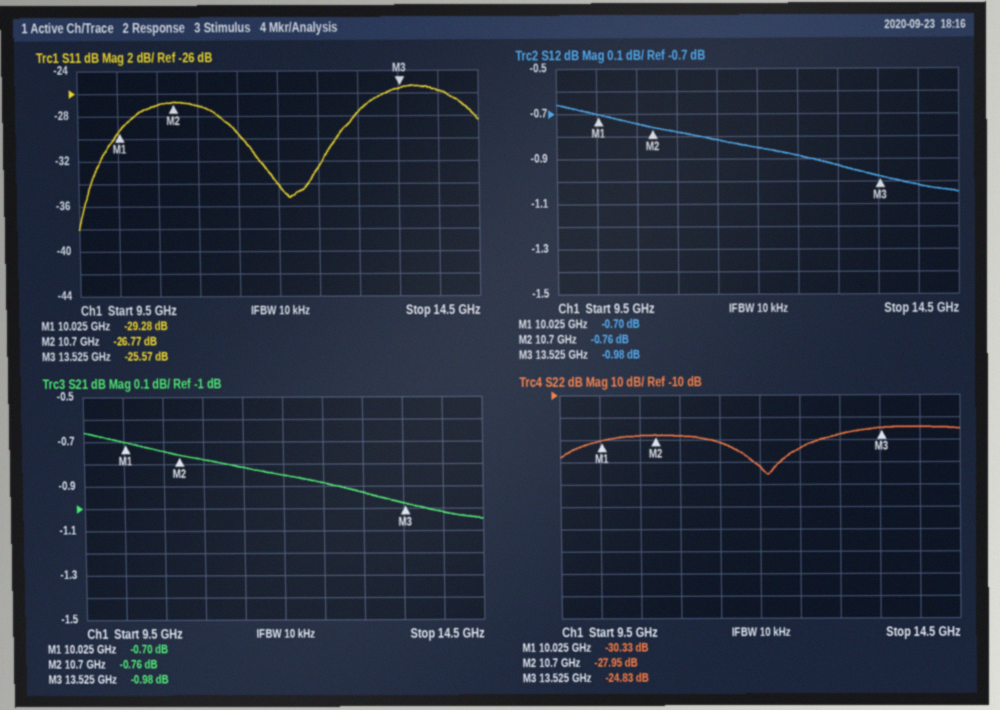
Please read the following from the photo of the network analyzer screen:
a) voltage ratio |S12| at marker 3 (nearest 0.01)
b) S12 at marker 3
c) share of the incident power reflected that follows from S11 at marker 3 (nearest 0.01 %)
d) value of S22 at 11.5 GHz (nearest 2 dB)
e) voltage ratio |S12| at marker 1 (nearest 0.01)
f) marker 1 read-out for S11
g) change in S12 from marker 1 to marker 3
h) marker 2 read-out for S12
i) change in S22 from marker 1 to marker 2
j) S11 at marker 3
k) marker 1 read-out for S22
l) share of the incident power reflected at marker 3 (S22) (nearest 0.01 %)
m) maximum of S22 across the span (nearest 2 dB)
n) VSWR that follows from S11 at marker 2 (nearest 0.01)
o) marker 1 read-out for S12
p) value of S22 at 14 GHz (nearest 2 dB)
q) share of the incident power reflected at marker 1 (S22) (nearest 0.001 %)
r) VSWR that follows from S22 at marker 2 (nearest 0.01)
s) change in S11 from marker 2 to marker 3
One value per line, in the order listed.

0.89
-0.98 dB
0.28 %
-32 dB
0.92
-29.28 dB
-0.28 dB
-0.76 dB
2.38 dB
-25.57 dB
-30.33 dB
0.33 %
-24 dB
1.10
-0.70 dB
-24 dB
0.093 %
1.08
1.20 dB
